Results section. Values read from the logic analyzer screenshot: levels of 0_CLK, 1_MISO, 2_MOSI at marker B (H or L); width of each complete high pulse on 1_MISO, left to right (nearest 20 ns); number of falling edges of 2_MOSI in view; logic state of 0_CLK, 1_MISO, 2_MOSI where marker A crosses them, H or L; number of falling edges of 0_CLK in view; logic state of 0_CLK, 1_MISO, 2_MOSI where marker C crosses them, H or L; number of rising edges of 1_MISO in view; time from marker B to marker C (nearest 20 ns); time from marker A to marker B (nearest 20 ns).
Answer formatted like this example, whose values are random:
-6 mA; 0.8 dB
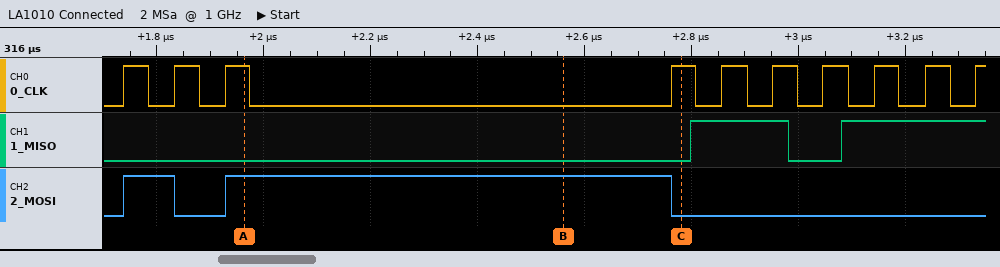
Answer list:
0_CLK=L, 1_MISO=L, 2_MOSI=H; 180 ns; 2; 0_CLK=H, 1_MISO=L, 2_MOSI=H; 9; 0_CLK=H, 1_MISO=L, 2_MOSI=L; 2; 220 ns; 600 ns
